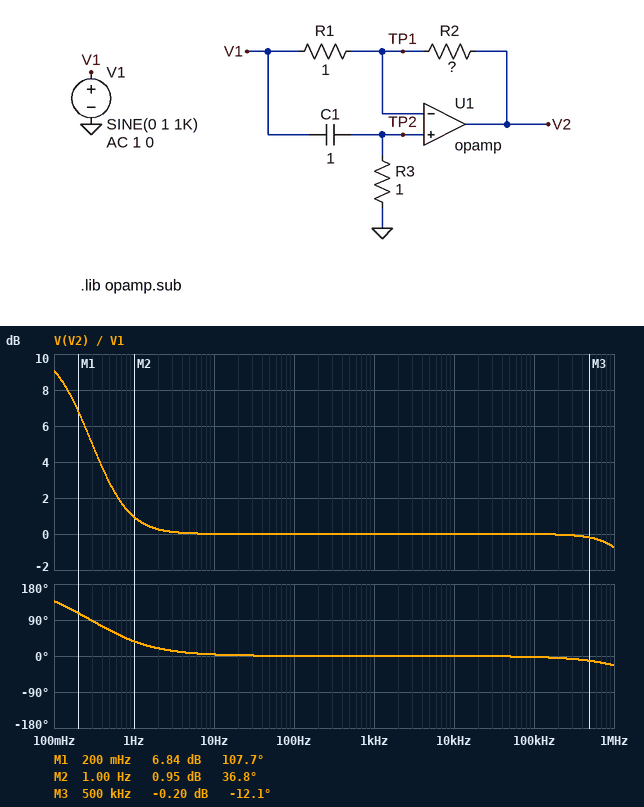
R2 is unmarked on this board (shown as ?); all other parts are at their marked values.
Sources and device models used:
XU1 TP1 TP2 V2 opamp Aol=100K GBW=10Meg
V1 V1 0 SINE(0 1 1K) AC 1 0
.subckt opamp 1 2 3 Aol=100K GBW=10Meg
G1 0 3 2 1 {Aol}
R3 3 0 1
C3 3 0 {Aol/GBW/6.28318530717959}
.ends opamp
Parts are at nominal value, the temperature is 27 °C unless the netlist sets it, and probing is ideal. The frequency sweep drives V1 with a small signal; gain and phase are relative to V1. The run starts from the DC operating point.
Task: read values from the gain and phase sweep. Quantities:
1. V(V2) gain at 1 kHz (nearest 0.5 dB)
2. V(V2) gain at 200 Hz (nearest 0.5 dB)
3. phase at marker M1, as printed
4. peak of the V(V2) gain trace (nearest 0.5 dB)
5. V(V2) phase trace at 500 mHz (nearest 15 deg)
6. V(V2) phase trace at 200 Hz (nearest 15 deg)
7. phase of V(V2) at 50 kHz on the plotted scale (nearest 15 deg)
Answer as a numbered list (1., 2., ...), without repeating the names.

1. 0 dB
2. 0 dB
3. 107.7 deg
4. 9.0 dB
5. 60 deg
6. 0 deg
7. 0 deg
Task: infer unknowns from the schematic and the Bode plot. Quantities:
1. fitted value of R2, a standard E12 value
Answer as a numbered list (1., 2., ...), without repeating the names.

1. 3.3 Ω
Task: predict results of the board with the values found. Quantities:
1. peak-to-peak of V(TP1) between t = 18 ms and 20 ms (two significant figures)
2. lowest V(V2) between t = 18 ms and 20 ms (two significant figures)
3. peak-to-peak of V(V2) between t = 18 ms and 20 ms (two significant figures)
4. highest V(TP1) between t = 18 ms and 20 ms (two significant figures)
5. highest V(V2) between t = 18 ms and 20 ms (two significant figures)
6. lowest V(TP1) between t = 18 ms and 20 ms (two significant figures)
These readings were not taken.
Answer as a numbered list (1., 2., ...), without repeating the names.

1. 2.0 V
2. -1.0 V
3. 2.0 V
4. 1.0 V
5. 1.0 V
6. -1.0 V
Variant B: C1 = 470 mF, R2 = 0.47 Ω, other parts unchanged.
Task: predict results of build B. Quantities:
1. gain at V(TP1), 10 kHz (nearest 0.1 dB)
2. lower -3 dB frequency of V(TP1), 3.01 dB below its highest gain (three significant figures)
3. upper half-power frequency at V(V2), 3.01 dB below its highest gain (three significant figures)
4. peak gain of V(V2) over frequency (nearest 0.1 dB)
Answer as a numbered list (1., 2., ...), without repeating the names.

1. 0 dB
2. 339 mHz
3. 6.80 MHz
4. 0 dB
